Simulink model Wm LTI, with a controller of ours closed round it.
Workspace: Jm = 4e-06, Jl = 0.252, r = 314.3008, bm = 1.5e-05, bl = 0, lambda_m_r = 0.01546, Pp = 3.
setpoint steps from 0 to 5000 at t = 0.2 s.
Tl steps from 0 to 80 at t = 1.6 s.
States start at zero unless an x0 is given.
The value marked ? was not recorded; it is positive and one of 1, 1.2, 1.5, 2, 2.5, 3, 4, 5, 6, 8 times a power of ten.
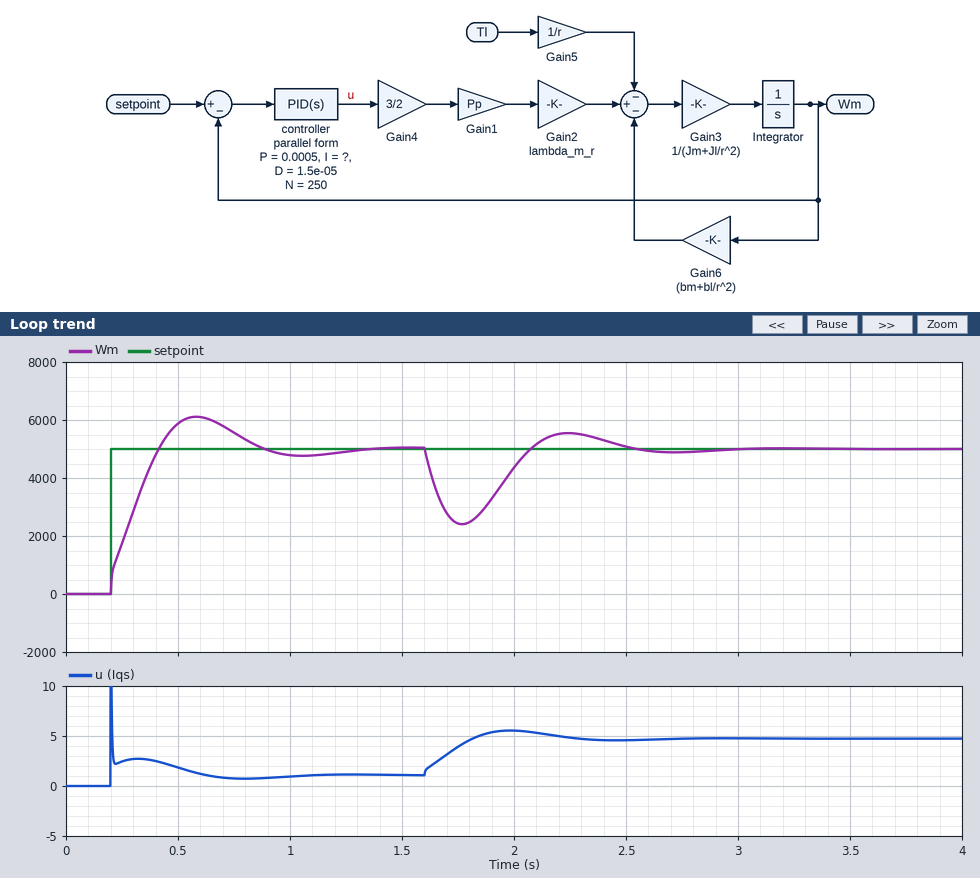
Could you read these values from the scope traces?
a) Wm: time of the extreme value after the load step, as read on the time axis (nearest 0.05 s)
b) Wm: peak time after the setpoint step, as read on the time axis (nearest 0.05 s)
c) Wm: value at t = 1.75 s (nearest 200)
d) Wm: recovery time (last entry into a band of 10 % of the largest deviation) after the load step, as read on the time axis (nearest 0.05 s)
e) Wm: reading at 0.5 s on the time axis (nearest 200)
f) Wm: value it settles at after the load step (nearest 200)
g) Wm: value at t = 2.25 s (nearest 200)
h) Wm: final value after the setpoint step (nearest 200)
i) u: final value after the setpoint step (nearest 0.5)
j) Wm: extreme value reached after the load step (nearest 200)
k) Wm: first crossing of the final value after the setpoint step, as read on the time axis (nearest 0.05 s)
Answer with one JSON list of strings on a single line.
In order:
["1.75 s", "0.60 s", "2400", "2.40 s", "5800", "5000", "5600", "5000", "1.0", "2400", "0.40 s"]
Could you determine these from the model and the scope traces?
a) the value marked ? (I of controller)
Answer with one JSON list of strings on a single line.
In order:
["0.006"]
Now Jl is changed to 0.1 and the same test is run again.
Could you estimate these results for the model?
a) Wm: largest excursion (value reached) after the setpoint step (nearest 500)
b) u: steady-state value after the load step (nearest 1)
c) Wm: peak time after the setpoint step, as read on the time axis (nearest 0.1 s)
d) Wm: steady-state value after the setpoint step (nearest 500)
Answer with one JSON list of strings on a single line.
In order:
["6000", "5", "0.5 s", "5000"]
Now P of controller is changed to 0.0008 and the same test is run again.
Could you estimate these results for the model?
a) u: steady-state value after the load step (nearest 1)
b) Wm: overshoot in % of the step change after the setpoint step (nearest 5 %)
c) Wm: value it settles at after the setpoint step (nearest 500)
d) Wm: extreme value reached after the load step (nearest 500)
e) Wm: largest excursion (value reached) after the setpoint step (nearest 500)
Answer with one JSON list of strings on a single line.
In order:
["5", "15 %", "5000", "3000", "5500"]
